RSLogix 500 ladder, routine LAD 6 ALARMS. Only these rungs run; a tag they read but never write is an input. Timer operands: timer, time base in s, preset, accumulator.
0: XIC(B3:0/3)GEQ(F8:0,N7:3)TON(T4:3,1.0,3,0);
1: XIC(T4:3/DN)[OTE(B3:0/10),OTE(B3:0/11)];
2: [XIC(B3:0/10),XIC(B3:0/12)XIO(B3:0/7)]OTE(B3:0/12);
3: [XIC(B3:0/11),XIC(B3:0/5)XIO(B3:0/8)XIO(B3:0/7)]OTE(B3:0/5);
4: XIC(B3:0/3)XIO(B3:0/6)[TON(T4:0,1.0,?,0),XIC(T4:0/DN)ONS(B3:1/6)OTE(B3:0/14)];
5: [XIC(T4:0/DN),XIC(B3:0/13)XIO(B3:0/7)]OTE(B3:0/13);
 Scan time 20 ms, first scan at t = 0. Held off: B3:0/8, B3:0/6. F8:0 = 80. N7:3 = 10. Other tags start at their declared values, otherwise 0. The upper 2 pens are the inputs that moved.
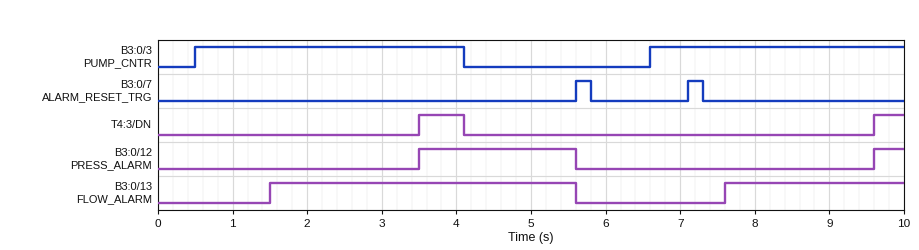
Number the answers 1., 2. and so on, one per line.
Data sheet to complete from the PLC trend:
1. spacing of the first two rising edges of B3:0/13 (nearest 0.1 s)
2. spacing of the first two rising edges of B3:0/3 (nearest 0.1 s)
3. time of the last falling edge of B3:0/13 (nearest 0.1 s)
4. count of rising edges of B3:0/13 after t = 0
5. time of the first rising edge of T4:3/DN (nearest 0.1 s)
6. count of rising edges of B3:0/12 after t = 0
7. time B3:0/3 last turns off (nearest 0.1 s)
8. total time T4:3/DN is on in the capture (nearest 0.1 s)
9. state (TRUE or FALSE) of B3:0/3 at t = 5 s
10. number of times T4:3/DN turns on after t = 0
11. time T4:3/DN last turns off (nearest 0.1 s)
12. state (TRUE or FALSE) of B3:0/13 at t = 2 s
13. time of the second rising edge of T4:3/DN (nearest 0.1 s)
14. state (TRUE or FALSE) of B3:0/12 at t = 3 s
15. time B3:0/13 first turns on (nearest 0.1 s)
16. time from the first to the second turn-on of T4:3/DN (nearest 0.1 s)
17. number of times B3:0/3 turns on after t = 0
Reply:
1. 6.1 s
2. 6.1 s
3. 5.6 s
4. 2
5. 3.5 s
6. 2
7. 4.1 s
8. 1.0 s
9. FALSE
10. 2
11. 4.1 s
12. TRUE
13. 9.6 s
14. FALSE
15. 1.5 s
16. 6.1 s
17. 2
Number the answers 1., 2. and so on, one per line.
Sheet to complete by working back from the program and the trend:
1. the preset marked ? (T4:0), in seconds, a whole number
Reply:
1. 1 s
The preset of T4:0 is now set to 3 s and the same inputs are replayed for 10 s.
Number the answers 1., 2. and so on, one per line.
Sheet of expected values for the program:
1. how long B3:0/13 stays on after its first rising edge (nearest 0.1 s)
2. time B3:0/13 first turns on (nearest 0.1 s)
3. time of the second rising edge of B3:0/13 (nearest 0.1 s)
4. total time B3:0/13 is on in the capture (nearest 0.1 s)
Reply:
1. 2.1 s
2. 3.5 s
3. 9.6 s
4. 2.5 s
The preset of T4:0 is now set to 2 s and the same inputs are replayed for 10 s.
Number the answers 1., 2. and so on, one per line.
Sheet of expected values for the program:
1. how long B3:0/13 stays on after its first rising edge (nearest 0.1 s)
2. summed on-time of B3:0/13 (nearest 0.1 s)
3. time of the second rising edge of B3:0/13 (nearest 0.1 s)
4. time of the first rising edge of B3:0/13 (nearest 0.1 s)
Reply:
1. 3.1 s
2. 4.5 s
3. 8.6 s
4. 2.5 s
